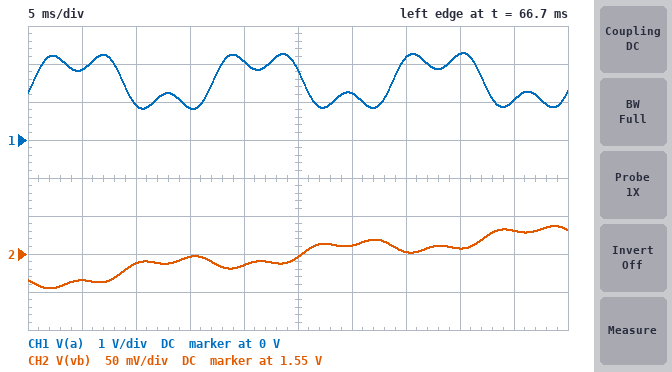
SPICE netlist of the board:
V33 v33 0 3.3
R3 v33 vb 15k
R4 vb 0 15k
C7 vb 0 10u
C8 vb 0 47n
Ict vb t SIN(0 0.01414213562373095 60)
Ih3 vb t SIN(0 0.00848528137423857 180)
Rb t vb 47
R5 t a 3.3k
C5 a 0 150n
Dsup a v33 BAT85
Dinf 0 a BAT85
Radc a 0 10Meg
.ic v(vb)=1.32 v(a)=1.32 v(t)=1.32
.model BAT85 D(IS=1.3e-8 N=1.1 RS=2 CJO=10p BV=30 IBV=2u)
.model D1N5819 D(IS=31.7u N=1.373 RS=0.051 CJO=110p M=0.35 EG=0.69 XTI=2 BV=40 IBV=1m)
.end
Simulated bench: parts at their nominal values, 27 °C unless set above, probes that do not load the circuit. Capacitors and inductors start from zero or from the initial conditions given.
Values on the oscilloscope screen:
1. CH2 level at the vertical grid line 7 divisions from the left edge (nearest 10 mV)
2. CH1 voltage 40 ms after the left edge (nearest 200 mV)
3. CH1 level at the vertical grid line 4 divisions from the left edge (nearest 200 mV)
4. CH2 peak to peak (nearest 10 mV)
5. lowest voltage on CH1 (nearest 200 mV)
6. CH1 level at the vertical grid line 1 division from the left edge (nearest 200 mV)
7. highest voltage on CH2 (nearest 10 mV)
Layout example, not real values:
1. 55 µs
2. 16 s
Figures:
1. 1.55 V
2. 2.2 V
3. 2.0 V
4. 80 mV
5. 800 mV
6. 1.8 V
7. 1.59 V
